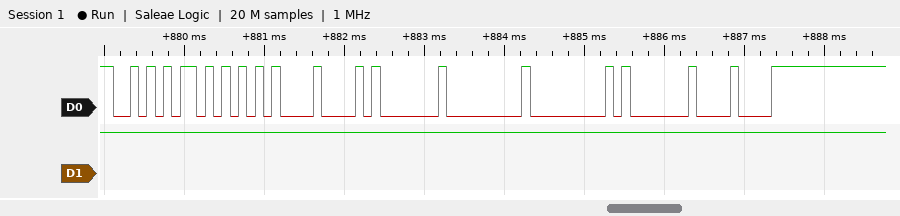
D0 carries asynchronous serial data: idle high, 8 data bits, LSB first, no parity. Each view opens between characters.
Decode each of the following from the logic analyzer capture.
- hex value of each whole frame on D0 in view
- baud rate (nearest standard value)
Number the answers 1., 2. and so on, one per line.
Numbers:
1. AA, 55, 08, 01, 00, 00, 01, 08
2. 9600 baud
